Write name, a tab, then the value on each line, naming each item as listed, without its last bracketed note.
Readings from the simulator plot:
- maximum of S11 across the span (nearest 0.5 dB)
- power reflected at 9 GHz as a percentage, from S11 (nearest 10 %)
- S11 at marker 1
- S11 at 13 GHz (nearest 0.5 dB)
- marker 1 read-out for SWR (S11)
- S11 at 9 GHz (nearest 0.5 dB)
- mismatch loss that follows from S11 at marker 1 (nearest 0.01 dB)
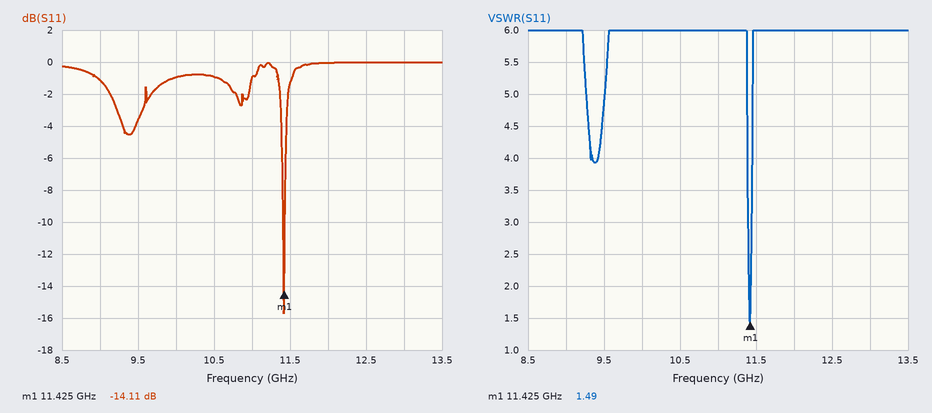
maximum of S11 across the span	0.0 dB
power reflected at 9 GHz as a percentage, from S11	80 %
S11 at marker 1	-14.11 dB
S11 at 13 GHz	0.0 dB
marker 1 read-out for SWR	1.49
S11 at 9 GHz	-1.0 dB
mismatch loss that follows from S11 at marker 1	0.17 dB
